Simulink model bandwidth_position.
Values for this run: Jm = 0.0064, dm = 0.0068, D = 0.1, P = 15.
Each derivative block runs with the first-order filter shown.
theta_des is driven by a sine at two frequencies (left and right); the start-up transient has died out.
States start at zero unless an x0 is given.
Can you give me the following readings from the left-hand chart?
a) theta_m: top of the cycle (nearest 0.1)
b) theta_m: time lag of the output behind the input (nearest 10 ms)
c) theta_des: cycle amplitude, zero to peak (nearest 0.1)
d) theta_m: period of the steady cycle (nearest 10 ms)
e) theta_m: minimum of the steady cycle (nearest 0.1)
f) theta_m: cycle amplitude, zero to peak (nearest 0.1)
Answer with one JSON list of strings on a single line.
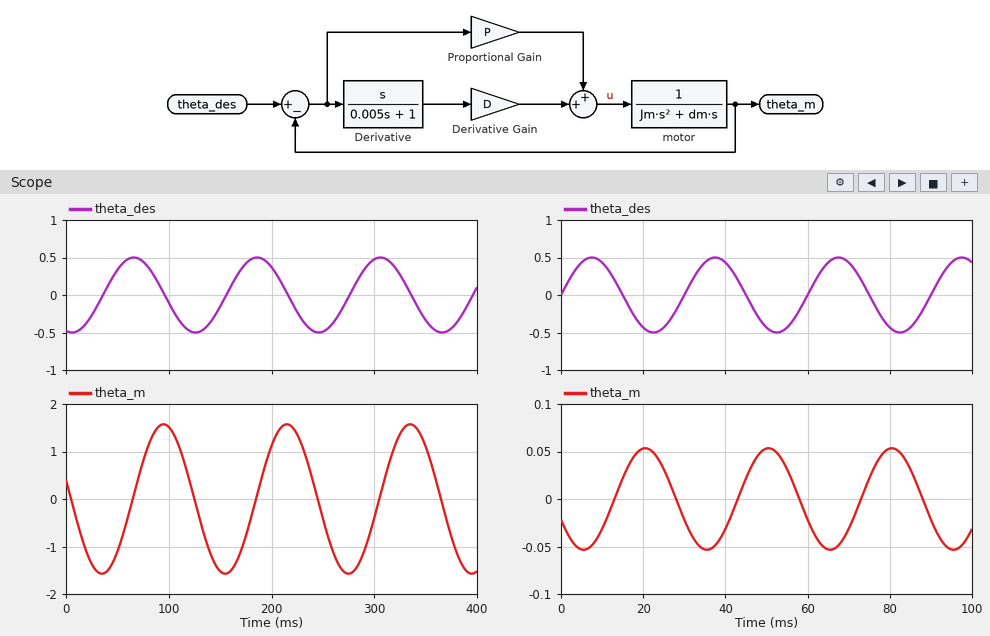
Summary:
["1.6", "30 ms", "0.5", "120 ms", "-1.6", "1.6"]
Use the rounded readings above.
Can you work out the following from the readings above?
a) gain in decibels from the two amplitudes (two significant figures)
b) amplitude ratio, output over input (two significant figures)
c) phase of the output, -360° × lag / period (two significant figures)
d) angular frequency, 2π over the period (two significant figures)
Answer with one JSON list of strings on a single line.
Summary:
["10 dB", "3.2", "-90°", "0.052 rad/ms"]
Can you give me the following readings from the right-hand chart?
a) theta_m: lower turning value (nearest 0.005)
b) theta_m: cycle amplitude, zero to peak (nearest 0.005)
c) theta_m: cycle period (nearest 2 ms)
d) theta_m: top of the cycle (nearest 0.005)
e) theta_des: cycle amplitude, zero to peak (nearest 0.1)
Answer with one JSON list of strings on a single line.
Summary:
["-0.055", "0.055", "30 ms", "0.055", "0.5"]
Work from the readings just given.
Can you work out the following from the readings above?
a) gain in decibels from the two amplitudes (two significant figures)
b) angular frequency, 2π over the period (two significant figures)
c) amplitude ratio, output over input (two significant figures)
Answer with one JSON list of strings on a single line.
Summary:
["-19 dB", "0.21 rad/ms", "0.11"]
